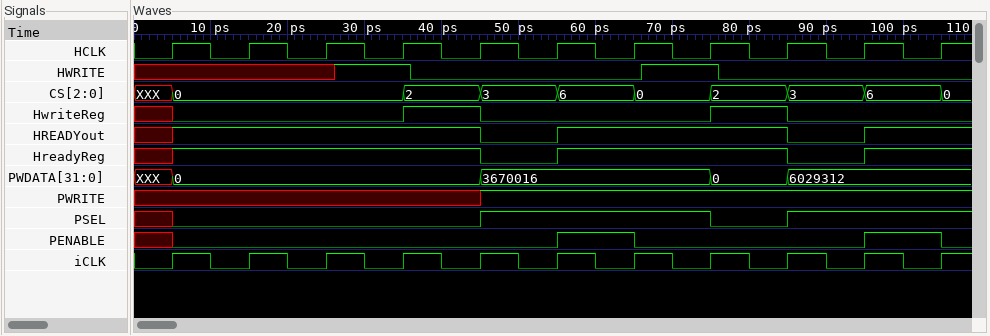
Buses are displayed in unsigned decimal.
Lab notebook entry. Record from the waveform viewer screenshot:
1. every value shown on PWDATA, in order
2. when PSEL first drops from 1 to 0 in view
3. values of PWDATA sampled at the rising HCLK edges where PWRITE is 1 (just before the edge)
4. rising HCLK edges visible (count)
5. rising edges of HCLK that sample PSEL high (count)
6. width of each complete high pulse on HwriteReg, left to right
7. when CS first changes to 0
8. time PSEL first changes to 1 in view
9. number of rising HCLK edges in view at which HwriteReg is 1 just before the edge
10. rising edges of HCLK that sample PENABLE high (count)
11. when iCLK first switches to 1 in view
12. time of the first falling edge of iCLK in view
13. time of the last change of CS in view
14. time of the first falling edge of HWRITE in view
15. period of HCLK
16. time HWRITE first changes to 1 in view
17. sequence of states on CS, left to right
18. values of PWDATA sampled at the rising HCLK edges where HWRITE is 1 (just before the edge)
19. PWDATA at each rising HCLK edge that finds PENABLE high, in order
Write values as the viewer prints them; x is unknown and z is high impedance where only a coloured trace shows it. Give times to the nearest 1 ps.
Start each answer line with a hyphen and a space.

- XXX, 0, 3670016, 0, 6029312
- 75 ps
- 3670016, 3670016, 3670016, 0, 6029312, 6029312
- 11
- 5
- 10 ps, 10 ps
- 5 ps
- 45 ps
- 2
- 2
- 5 ps
- 10 ps
- 105 ps
- 36 ps
- 10 ps
- 26 ps
- XXX, 0, 2, 3, 6, 0, 2, 3, 6, 0
- 0, 3670016
- 3670016, 6029312
